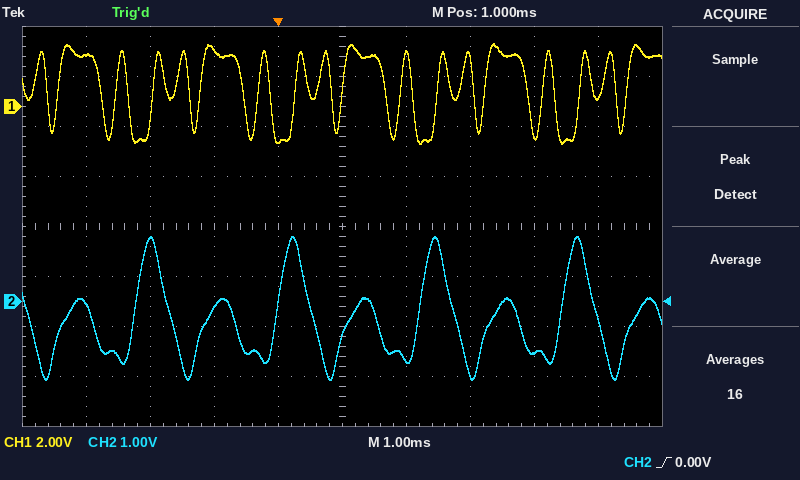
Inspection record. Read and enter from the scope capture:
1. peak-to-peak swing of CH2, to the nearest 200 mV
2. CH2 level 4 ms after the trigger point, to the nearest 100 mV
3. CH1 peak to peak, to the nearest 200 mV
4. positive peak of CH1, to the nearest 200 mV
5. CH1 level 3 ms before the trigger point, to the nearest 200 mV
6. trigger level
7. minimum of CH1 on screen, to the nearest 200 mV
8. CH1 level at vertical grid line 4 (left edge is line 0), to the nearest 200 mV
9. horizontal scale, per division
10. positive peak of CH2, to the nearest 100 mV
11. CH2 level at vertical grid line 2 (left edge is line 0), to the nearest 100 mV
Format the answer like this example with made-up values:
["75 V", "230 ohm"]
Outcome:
["2.8 V", "-1.0 V", "4.0 V", "2.6 V", "2.0 V", "0.00 V", "-1.4 V", "-1.4 V", "1 ms", "1.3 V", "1.2 V"]
